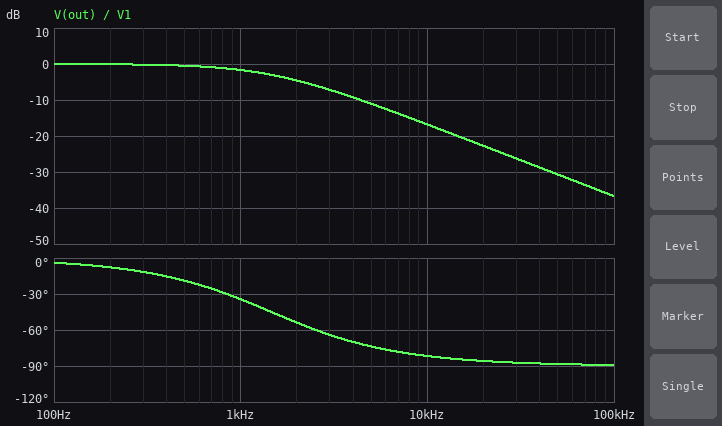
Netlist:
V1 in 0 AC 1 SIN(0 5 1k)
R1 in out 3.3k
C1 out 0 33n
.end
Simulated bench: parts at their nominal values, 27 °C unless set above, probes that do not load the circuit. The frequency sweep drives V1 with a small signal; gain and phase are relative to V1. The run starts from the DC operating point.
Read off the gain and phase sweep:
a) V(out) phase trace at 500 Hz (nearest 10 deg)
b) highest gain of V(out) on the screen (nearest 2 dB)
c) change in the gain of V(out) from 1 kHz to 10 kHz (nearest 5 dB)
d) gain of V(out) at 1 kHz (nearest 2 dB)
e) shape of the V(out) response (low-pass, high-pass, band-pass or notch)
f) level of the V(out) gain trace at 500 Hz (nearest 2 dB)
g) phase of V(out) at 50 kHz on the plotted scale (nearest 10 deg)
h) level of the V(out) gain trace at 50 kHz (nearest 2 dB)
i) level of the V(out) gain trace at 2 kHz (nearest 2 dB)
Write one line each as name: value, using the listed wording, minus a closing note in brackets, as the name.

V(out) phase trace at 500 Hz: -20 deg
highest gain of V(out) on the screen: 0 dB
change in the gain of V(out) from 1 kHz to 10 kHz: -15 dB
gain of V(out) at 1 kHz: -2 dB
shape of the V(out) response: low-pass
level of the V(out) gain trace at 500 Hz: 0 dB
phase of V(out) at 50 kHz on the plotted scale: -90 deg
level of the V(out) gain trace at 50 kHz: -30 dB
level of the V(out) gain trace at 2 kHz: -4 dB
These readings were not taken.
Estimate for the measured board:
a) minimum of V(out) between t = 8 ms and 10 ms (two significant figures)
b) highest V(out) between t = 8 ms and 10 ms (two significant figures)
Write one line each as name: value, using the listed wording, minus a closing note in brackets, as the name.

minimum of V(out) between t = 8 ms and 10 ms: -4.1 V
highest V(out) between t = 8 ms and 10 ms: 4.1 V
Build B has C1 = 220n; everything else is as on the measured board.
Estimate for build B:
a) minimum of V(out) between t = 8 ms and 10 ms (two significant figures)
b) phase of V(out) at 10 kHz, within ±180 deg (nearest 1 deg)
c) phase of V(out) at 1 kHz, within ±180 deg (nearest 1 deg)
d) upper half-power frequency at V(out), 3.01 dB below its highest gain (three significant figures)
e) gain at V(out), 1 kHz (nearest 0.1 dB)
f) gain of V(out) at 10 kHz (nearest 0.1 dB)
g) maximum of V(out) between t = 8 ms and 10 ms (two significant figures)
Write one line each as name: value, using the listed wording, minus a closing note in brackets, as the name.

minimum of V(out) between t = 8 ms and 10 ms: -1.1 V
phase of V(out) at 10 kHz, within ±180 deg: -89 deg
phase of V(out) at 1 kHz, within ±180 deg: -78 deg
upper half-power frequency at V(out), 3.01 dB below its highest gain: 219 Hz
gain at V(out), 1 kHz: -13.4 dB
gain of V(out) at 10 kHz: -33.2 dB
maximum of V(out) between t = 8 ms and 10 ms: 1.1 V
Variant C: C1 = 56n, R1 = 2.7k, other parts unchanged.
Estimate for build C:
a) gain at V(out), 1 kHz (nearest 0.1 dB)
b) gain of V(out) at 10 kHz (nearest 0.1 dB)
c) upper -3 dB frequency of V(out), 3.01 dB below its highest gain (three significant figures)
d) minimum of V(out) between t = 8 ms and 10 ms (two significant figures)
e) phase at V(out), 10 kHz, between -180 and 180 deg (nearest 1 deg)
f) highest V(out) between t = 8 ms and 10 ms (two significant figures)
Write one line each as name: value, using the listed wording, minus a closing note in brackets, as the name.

gain at V(out), 1 kHz: -2.8 dB
gain of V(out) at 10 kHz: -19.6 dB
upper -3 dB frequency of V(out), 3.01 dB below its highest gain: 1.05 kHz
minimum of V(out) between t = 8 ms and 10 ms: -3.6 V
phase at V(out), 10 kHz, between -180 and 180 deg: -84 deg
highest V(out) between t = 8 ms and 10 ms: 3.6 V
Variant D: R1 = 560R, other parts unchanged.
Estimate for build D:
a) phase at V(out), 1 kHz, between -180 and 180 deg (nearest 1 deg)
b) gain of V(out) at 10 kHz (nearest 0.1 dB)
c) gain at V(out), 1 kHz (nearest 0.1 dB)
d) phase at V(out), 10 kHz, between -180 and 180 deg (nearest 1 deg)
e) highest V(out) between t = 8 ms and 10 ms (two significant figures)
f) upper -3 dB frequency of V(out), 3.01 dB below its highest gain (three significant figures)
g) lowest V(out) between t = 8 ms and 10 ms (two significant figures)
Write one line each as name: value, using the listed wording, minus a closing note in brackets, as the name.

phase at V(out), 1 kHz, between -180 and 180 deg: -7 deg
gain of V(out) at 10 kHz: -3.7 dB
gain at V(out), 1 kHz: -0.1 dB
phase at V(out), 10 kHz, between -180 and 180 deg: -49 deg
highest V(out) between t = 8 ms and 10 ms: 5.0 V
upper -3 dB frequency of V(out), 3.01 dB below its highest gain: 8.61 kHz
lowest V(out) between t = 8 ms and 10 ms: -5.0 V
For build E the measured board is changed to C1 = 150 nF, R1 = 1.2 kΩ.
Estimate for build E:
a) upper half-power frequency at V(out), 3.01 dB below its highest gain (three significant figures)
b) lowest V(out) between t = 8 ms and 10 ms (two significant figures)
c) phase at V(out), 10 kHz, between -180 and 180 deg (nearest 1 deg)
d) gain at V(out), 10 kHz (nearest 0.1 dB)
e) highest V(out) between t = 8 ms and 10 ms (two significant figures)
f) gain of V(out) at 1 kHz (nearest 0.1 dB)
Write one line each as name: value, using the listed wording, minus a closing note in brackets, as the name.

upper half-power frequency at V(out), 3.01 dB below its highest gain: 884 Hz
lowest V(out) between t = 8 ms and 10 ms: -3.3 V
phase at V(out), 10 kHz, between -180 and 180 deg: -85 deg
gain at V(out), 10 kHz: -21.1 dB
highest V(out) between t = 8 ms and 10 ms: 3.3 V
gain of V(out) at 1 kHz: -3.6 dB
